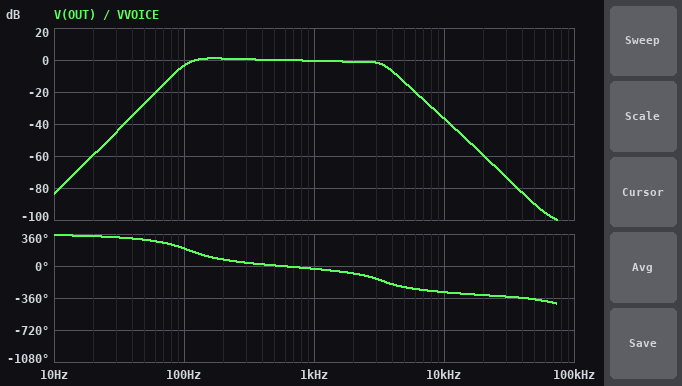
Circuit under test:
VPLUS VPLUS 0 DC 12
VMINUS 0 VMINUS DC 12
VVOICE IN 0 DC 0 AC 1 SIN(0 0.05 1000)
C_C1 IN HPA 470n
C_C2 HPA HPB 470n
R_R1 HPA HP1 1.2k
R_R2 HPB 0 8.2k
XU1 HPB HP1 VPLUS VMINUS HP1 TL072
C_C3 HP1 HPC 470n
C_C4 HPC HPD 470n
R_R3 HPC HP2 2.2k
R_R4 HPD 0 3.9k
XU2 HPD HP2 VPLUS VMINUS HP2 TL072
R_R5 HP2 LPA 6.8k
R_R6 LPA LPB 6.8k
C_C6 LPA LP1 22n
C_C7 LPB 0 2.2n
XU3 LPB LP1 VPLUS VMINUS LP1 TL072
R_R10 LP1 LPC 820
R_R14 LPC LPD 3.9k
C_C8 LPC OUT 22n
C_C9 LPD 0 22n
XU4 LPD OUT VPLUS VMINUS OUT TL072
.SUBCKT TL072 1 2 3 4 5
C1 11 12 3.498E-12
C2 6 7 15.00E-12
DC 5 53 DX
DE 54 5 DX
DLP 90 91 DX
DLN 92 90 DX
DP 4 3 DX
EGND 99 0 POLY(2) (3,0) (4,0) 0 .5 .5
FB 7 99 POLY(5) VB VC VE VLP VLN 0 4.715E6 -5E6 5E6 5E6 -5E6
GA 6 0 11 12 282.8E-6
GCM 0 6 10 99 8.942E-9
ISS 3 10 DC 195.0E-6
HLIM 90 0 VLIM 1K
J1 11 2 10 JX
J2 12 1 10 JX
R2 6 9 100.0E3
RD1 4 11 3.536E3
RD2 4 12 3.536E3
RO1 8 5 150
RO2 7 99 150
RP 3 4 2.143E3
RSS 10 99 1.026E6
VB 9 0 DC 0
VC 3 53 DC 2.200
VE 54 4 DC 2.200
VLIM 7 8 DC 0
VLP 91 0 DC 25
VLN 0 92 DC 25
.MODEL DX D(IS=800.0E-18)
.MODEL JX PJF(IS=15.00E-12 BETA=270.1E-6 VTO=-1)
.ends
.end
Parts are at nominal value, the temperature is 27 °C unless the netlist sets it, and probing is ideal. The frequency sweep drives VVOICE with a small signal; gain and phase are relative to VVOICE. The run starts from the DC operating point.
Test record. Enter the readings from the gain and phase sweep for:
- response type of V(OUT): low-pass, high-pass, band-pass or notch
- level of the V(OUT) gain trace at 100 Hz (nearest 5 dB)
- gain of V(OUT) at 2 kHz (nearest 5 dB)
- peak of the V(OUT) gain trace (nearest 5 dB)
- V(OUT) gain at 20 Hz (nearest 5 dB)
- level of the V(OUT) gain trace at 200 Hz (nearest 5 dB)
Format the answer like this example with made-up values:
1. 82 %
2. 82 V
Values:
1. band-pass
2. -5 dB
3. 0 dB
4. 0 dB
5. -60 dB
6. 0 dB
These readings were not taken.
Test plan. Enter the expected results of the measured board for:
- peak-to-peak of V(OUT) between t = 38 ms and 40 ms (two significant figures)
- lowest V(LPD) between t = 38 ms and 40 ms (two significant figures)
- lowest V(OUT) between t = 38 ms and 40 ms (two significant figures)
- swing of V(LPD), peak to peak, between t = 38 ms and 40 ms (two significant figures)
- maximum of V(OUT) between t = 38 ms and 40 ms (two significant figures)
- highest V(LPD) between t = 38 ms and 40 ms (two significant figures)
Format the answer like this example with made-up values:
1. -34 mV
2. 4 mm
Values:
1. 95 mV
2. -47 mV
3. -47 mV
4. 95 mV
5. 47 mV
6. 47 mV
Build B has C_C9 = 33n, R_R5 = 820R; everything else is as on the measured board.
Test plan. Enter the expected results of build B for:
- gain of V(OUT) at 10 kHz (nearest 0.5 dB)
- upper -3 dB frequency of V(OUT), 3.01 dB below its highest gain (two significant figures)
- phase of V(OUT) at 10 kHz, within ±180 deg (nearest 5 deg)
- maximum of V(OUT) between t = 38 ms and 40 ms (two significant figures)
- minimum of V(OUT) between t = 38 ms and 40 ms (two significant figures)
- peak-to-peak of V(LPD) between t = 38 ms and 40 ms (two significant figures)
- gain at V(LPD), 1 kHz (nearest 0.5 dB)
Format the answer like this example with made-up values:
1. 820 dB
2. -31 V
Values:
1. -22.5 dB
2. 910 Hz
3. 135 deg
4. 38 mV
5. -38 mV
6. 76 mV
7. -2.5 dB
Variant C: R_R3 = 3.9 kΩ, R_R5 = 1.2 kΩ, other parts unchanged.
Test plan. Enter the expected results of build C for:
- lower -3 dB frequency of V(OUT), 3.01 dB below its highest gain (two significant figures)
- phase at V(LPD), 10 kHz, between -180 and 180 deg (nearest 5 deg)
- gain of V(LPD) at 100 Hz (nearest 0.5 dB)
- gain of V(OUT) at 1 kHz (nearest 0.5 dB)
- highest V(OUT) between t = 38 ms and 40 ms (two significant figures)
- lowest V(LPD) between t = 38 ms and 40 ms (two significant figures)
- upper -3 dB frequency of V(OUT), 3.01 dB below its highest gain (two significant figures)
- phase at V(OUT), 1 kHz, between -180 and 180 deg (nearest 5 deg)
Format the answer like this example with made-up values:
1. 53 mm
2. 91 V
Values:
1. 100 Hz
2. 115 deg
3. -3.5 dB
4. -1.0 dB
5. 44 mV
6. -44 mV
7. 1.8 kHz
8. -25 deg
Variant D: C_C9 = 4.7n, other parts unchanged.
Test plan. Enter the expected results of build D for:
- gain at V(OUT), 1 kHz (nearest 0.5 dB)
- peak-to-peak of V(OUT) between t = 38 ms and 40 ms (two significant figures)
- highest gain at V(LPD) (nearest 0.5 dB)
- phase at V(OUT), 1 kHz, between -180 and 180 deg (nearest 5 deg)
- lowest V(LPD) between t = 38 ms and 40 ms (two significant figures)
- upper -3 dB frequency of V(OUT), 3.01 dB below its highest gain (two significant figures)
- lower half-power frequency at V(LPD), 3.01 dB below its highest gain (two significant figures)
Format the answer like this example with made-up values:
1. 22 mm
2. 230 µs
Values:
1. 0.5 dB
2. 110 mV
3. 4.5 dB
4. -5 deg
5. -54 mV
6. 4.0 kHz
7. 1.6 kHz
